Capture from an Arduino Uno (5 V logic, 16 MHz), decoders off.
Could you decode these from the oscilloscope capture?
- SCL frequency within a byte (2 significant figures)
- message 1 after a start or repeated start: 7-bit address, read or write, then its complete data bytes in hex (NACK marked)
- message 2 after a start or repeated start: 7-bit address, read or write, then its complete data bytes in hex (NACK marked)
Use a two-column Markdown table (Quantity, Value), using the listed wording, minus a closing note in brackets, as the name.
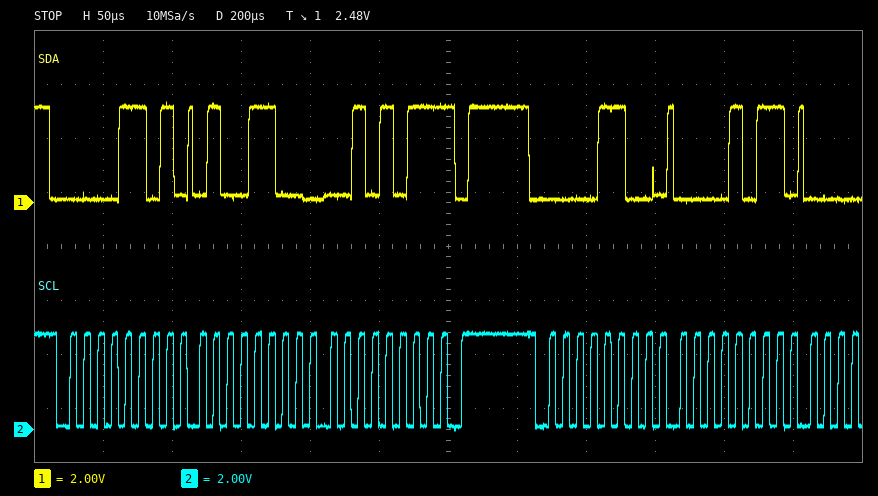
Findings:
| Quantity | Value |
|---|---|
| SCL frequency within a byte | 100 kHz |
| message 1 after a start or repeated start: 7-bit address, read or write, then its complete data bytes in hex | 0x06 read: 4C 2B NACK |
| message 2 after a start or repeated start: 7-bit address, read or write, then its complete data bytes in hex | 0x06 write: 0B |
